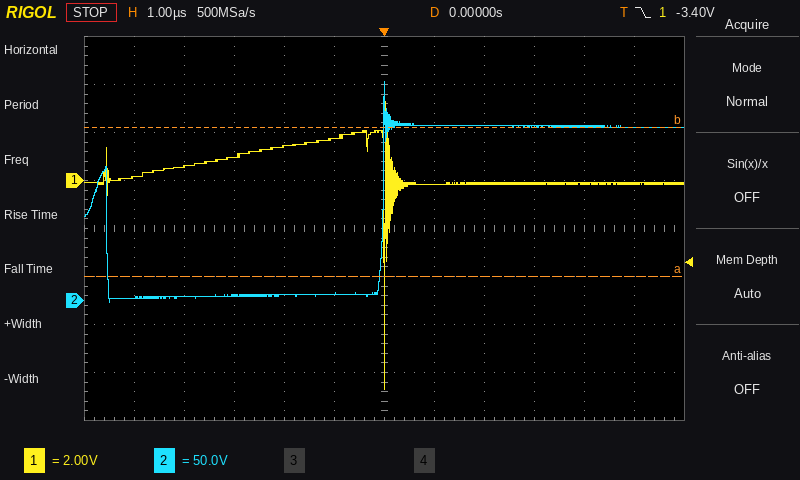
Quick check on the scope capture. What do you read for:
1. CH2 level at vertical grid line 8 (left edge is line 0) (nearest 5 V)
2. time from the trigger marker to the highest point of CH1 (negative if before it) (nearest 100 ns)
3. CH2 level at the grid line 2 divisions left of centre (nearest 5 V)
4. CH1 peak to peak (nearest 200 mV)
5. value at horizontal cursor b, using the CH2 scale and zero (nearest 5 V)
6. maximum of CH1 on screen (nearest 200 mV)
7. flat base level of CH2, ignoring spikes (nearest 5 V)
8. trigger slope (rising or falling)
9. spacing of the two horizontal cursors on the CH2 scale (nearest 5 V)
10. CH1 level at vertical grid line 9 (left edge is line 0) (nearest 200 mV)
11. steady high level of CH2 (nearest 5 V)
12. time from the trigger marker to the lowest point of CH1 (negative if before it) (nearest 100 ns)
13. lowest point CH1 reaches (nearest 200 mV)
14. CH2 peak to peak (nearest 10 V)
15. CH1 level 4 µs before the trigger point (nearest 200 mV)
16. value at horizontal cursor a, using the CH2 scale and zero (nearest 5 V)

180 V
0.0 µs
5 V
12.0 V
180 V
3.2 V
5 V
falling
155 V
-200 mV
180 V
0.0 µs
-8.8 V
230 V
600 mV
25 V
